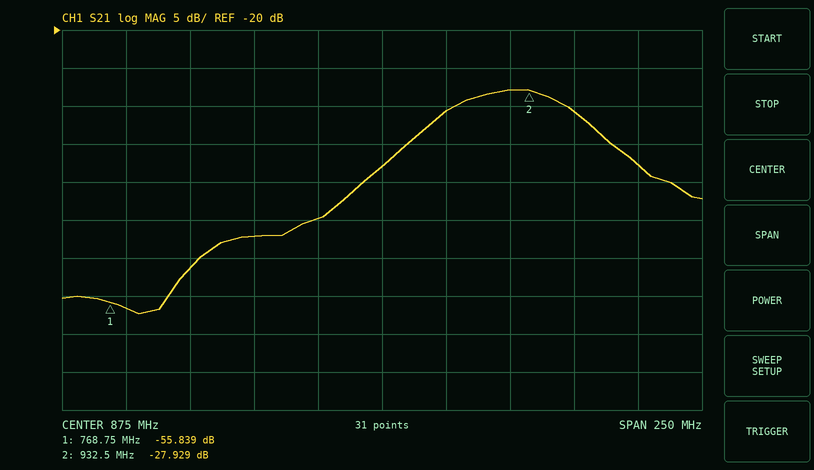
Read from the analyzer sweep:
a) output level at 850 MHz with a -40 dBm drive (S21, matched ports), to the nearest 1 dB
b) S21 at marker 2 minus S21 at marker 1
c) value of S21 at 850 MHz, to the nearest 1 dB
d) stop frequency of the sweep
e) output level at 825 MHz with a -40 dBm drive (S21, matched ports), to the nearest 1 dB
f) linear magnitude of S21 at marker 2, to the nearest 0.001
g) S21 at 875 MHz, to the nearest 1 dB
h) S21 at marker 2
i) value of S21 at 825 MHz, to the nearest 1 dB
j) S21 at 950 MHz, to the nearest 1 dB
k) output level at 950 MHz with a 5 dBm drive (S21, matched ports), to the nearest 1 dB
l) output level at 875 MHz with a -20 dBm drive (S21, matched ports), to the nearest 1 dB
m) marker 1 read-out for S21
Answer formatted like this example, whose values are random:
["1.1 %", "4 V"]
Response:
["-85 dBm", "27.910 dB", "-45 dB", "1 GHz", "-87 dBm", "0.040", "-38 dB", "-27.929 dB", "-47 dB", "-31 dB", "-26 dBm", "-58 dBm", "-55.839 dB"]
